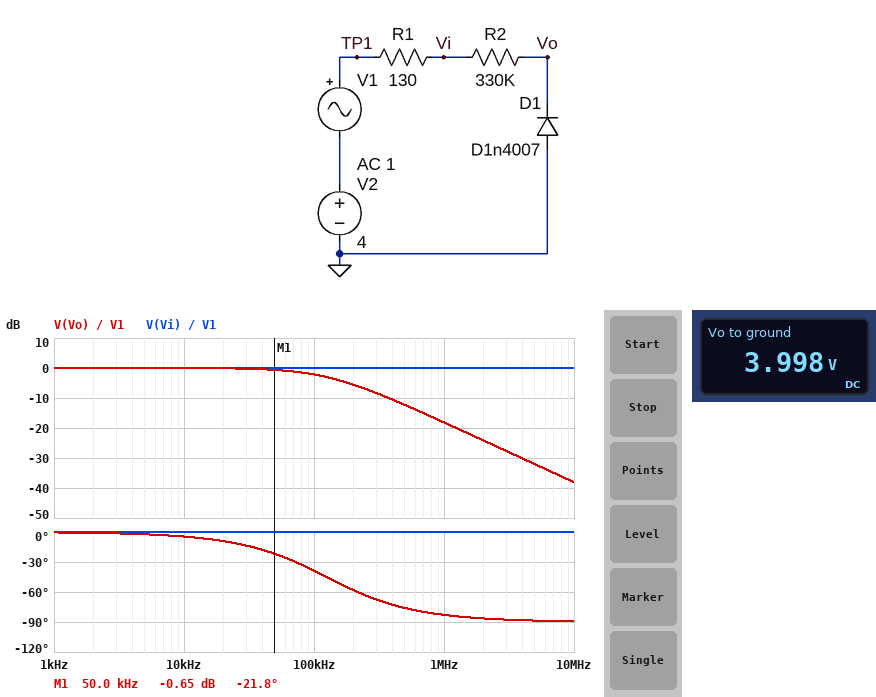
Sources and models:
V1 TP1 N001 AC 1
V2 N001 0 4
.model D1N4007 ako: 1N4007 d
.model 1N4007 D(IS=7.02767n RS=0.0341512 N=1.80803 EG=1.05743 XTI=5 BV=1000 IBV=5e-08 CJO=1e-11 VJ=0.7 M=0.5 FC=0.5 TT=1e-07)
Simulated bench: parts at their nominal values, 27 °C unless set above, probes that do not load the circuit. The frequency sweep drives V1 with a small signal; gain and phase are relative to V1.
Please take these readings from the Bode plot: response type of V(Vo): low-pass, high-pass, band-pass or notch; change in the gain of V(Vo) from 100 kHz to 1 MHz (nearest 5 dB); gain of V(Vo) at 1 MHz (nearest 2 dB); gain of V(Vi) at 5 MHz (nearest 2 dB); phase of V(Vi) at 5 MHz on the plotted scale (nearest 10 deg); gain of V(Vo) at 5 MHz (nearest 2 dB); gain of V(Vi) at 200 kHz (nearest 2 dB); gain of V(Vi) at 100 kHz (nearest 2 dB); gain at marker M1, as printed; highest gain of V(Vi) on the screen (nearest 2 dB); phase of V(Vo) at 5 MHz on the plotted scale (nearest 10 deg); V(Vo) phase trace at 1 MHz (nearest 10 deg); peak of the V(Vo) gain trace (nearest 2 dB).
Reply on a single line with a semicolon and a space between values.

low-pass; -15 dB; -18 dB; 0 dB; 0 deg; -32 dB; 0 dB; 0 dB; -0.65 dB; 0 dB; -90 deg; -80 deg; 0 dB
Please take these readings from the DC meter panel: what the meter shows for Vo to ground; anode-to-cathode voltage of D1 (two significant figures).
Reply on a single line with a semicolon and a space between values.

3.998 V; -4.0 V
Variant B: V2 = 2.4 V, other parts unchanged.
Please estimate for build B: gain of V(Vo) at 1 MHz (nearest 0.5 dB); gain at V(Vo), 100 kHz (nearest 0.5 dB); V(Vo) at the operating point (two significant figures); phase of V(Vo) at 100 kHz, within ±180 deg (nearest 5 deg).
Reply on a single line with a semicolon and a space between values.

-20.0 dB; -3.0 dB; 2.4 V; -45 deg
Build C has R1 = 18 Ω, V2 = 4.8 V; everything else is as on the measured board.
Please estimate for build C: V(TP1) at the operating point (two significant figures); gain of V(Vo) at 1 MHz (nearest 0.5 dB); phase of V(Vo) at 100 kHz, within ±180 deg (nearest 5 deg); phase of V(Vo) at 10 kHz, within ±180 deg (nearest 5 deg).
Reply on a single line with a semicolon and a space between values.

4.8 V; -17.5 dB; -35 deg; -5 deg
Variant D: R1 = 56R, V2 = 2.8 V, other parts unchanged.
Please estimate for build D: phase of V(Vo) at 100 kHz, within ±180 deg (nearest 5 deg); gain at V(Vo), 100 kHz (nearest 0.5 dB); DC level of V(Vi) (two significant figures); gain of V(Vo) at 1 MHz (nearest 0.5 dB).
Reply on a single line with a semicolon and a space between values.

-45 deg; -2.5 dB; 2.8 V; -19.5 dB
